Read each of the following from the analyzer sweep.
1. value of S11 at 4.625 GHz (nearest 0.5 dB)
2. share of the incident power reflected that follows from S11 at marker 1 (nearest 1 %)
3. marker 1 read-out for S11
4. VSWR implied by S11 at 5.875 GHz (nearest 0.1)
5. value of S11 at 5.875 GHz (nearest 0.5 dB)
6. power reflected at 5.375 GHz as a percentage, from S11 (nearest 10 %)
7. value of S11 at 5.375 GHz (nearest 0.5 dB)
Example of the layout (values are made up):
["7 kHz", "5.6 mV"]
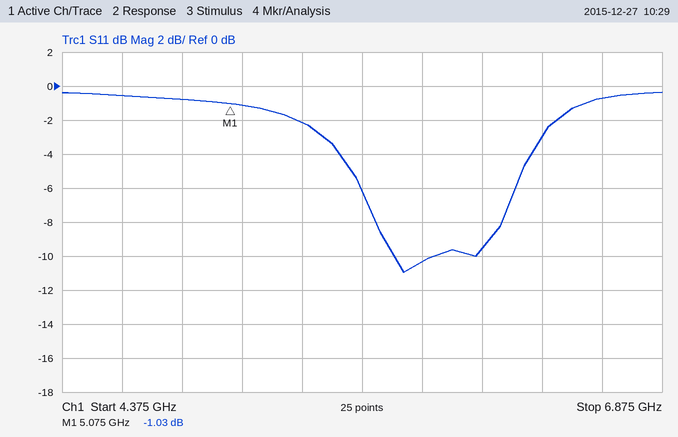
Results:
["-0.5 dB", "79 %", "-1.03 dB", "1.9", "-10.5 dB", "60 %", "-2.0 dB"]
